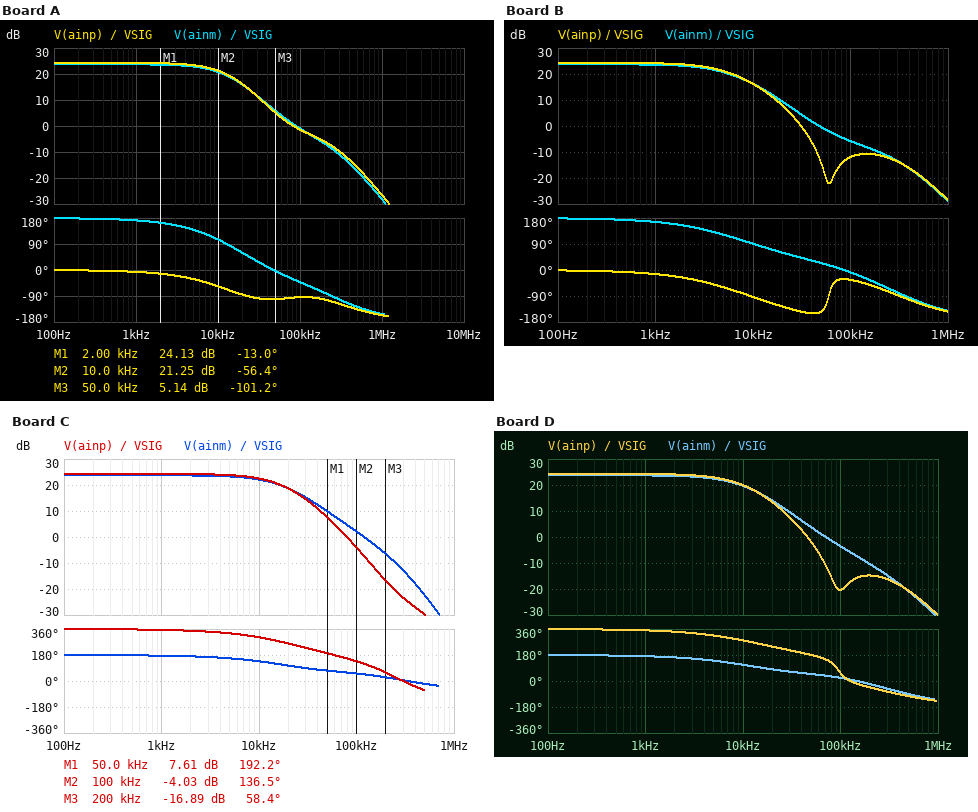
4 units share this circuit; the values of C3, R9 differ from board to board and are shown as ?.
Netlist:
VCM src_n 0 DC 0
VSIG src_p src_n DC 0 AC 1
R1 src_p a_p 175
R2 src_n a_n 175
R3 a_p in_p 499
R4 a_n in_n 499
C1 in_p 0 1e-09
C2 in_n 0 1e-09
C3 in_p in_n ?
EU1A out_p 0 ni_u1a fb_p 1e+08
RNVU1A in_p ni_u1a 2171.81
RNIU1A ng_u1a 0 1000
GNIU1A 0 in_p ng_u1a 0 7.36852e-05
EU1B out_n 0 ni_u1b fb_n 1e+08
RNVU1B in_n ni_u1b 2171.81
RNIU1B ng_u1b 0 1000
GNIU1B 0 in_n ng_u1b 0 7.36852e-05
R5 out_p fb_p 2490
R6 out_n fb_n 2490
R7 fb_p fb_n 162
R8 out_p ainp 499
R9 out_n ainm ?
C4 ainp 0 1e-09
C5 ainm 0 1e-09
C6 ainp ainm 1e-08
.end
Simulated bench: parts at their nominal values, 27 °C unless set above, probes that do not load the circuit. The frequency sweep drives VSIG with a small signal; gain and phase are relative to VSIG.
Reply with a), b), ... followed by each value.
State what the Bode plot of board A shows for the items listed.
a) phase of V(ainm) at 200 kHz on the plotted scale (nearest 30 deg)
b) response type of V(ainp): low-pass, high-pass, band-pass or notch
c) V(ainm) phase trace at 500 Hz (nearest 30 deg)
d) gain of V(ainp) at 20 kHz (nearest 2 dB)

a) -90 deg
b) low-pass
c) 180 deg
d) 16 dB
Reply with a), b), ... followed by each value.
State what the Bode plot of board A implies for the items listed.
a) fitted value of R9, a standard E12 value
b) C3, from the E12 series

a) 680 Ω
b) 5.6 nF
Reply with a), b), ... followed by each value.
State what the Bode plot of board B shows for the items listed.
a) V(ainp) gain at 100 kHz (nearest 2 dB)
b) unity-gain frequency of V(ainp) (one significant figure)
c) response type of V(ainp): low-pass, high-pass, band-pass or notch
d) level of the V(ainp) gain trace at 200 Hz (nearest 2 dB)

a) -12 dB
b) 30 kHz
c) low-pass
d) 24 dB
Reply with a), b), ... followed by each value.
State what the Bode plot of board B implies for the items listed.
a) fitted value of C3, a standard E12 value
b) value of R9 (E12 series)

a) 22 nF
b) 330 Ω
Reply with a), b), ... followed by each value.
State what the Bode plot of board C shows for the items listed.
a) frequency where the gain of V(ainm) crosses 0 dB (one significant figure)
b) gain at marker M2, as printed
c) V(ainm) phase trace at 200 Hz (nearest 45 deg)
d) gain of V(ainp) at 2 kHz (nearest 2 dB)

a) 100 kHz
b) -4.03 dB
c) 180 deg
d) 24 dB
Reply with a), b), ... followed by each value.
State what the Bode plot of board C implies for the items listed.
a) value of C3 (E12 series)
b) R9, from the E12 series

a) 4.7 nF
b) 270 Ω
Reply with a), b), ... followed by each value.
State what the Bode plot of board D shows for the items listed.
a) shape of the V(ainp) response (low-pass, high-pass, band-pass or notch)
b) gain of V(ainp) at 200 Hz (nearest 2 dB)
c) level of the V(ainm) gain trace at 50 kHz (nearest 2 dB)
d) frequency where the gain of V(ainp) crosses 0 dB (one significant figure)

a) low-pass
b) 24 dB
c) 4 dB
d) 50 kHz
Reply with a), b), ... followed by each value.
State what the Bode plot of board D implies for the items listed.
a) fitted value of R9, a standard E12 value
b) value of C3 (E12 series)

a) 270 Ω
b) 12 nF
